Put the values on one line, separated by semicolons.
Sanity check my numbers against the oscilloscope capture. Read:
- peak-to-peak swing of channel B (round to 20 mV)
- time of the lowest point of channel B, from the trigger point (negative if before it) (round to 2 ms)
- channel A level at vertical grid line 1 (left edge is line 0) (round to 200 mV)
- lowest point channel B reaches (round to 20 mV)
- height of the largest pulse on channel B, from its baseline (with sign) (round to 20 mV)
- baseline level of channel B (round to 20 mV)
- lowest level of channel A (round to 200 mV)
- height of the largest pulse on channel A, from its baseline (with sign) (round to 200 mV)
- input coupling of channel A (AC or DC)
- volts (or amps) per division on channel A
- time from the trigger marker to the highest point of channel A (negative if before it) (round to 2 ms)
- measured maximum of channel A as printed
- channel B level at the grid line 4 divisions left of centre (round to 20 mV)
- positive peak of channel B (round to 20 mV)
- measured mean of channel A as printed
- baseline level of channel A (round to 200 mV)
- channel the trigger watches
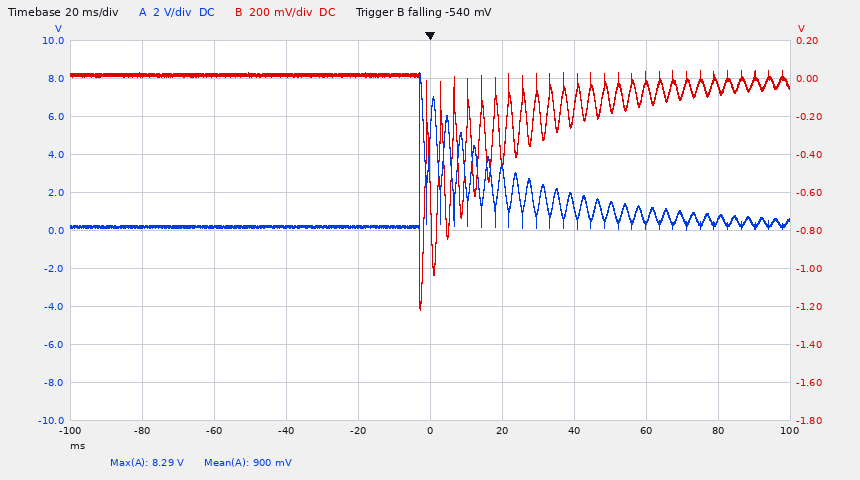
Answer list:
1.26 V; -2 ms; 200 mV; -1.22 V; -1.24 V; 20 mV; 0.0 V; +8.0 V; DC; 2 V; -2 ms; 8.29 V; 20 mV; 40 mV; 900 mV; 200 mV; channel B
